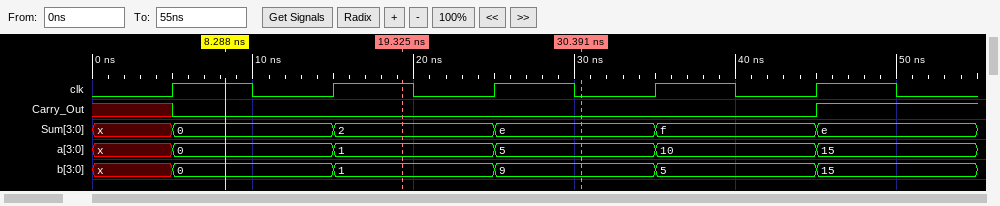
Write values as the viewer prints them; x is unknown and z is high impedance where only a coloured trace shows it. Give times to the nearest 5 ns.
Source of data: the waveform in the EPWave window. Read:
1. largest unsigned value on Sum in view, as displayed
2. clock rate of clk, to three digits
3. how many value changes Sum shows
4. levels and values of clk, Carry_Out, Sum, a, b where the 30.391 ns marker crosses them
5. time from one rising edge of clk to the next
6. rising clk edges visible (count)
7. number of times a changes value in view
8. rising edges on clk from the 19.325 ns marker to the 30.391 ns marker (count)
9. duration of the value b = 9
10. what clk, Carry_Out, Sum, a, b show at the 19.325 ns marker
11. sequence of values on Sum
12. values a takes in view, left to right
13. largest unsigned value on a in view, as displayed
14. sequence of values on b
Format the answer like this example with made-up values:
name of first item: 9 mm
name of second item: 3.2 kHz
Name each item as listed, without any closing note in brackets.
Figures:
largest unsigned value on Sum in view, as displayed: f
clock rate of clk, to three digits: 100 MHz
how many value changes Sum shows: 5
levels and values of clk, Carry_Out, Sum, a, b where the 30.391 ns marker crosses them: clk=0, Carry_Out=0, Sum=e, a=5, b=9
time from one rising edge of clk to the next: 10 ns
rising clk edges visible: 5
number of times a changes value in view: 5
rising edges on clk from the 19.325 ns marker to the 30.391 ns marker: 1
duration of the value b = 9: 10 ns
what clk, Carry_Out, Sum, a, b show at the 19.325 ns marker: clk=1, Carry_Out=0, Sum=2, a=1, b=1
sequence of values on Sum: x, 0, 2, e, f, e
values a takes in view, left to right: x, 0, 1, 5, 10, 15
largest unsigned value on a in view, as displayed: 15
sequence of values on b: x, 0, 1, 9, 5, 15
